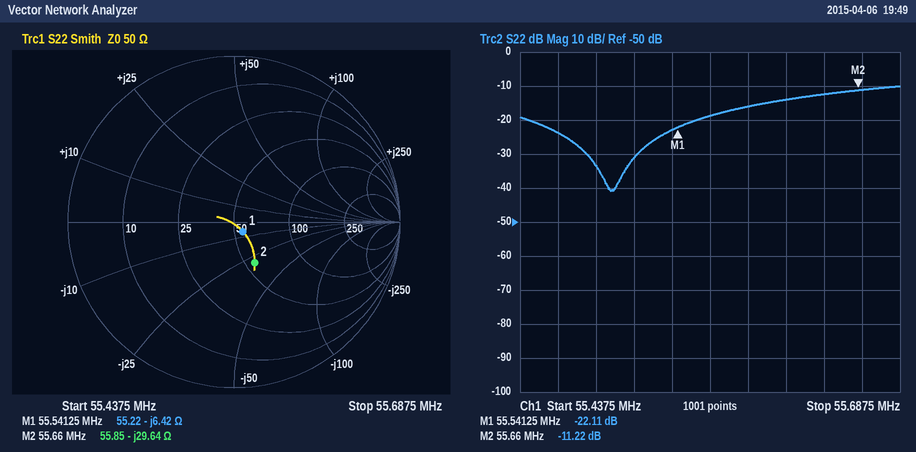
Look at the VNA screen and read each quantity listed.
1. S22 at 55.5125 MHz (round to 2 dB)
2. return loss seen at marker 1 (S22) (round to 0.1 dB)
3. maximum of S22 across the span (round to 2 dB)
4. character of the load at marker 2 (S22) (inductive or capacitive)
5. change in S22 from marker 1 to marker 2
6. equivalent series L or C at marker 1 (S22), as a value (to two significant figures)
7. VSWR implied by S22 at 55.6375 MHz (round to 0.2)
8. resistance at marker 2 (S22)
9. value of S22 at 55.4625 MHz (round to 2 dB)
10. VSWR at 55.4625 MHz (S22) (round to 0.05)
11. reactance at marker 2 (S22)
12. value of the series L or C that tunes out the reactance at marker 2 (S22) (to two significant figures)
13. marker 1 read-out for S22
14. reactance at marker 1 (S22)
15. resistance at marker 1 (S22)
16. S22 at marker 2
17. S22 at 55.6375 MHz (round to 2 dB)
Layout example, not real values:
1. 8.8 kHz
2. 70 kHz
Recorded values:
1. -32 dB
2. 22.1 dB
3. -10 dB
4. capacitive
5. 10.89 dB
6. 450 pF
7. 1.6
8. 55.85 Ω
9. -24 dB
10. 1.15
11. -29.64 Ω
12. 85 nH
13. -22.11 dB
14. -6.42 Ω
15. 55.22 Ω
16. -11.22 dB
17. -12 dB
